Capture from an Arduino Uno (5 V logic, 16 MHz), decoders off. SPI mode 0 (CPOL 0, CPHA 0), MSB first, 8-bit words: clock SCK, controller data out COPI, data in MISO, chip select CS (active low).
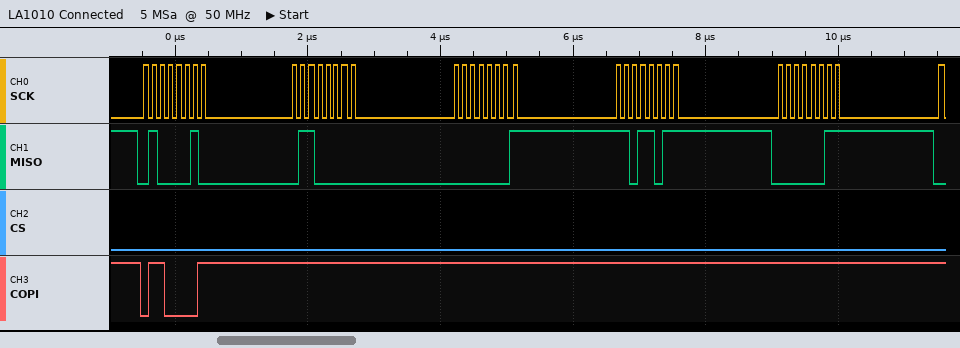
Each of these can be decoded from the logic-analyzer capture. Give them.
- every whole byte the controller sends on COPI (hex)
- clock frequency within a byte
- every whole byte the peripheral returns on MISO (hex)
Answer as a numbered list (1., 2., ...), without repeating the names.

1. 61 FF FF FF FF
2. 8 MHz
3. 42 60 01 DB 03
